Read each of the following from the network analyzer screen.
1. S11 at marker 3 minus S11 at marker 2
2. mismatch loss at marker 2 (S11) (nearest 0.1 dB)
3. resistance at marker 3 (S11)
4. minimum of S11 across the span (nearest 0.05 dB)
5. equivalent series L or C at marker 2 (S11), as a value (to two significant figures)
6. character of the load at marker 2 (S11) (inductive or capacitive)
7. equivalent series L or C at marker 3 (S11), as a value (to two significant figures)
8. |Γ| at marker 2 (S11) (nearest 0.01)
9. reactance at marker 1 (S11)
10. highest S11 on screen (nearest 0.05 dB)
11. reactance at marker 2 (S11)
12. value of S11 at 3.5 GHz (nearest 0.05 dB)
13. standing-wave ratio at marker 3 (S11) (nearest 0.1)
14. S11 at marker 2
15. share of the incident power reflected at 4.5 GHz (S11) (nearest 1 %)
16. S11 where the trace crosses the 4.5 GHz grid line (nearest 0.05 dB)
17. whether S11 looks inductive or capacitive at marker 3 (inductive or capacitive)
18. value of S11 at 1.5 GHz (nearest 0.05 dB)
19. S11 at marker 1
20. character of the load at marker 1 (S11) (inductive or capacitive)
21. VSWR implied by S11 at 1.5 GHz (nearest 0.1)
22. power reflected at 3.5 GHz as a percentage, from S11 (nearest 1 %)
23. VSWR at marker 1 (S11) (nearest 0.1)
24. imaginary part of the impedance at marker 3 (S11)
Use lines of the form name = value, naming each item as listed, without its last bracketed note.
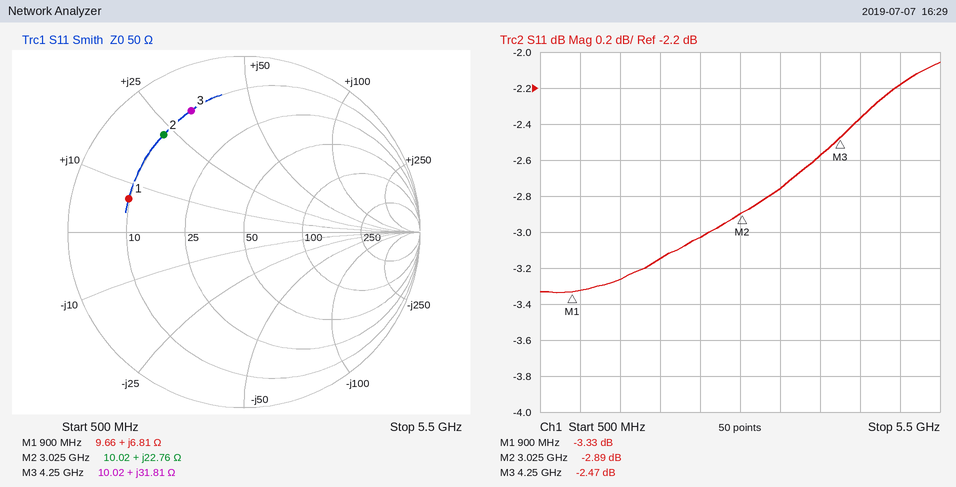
S11 at marker 3 minus S11 at marker 2 = 0.42 dB
mismatch loss at marker 2 (S11) = 3.1 dB
resistance at marker 3 = 10.02 Ω
minimum of S11 across the span = -3.35 dB
equivalent series L or C at marker 2 (S11), as a value = 1.2 nH
character of the load at marker 2 (S11) = inductive
equivalent series L or C at marker 3 (S11), as a value = 1.2 nH
|Γ| at marker 2 (S11) = 0.72
reactance at marker 1 = +6.81 Ω
highest S11 on screen = -2.05 dB
reactance at marker 2 = +22.76 Ω
value of S11 at 3.5 GHz = -2.75 dB
standing-wave ratio at marker 3 (S11) = 7.1
S11 at marker 2 = -2.89 dB
share of the incident power reflected at 4.5 GHz (S11) = 58 %
S11 where the trace crosses the 4.5 GHz grid line = -2.35 dB
whether S11 looks inductive or capacitive at marker 3 = inductive
value of S11 at 1.5 GHz = -3.25 dB
S11 at marker 1 = -3.33 dB
character of the load at marker 1 (S11) = inductive
VSWR implied by S11 at 1.5 GHz = 5.4
power reflected at 3.5 GHz as a percentage, from S11 = 53 %
VSWR at marker 1 (S11) = 5.3
imaginary part of the impedance at marker 3 = +31.81 Ω
